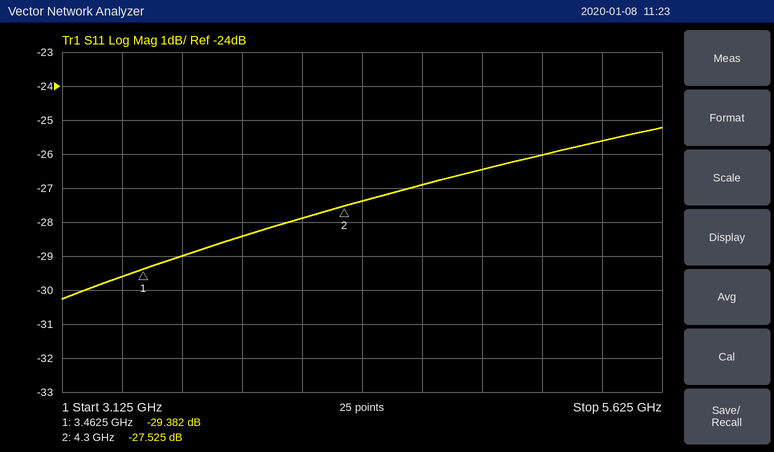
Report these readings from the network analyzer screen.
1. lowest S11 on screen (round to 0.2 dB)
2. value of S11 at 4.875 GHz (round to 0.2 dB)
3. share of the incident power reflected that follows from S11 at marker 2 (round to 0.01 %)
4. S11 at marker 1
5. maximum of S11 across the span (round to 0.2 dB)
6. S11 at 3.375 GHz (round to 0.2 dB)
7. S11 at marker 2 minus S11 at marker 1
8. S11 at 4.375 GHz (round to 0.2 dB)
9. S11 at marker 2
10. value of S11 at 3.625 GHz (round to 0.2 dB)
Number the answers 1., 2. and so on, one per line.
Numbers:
1. -30.2 dB
2. -26.4 dB
3. 0.18 %
4. -29.382 dB
5. -25.2 dB
6. -29.6 dB
7. 1.857 dB
8. -27.4 dB
9. -27.525 dB
10. -29.0 dB
